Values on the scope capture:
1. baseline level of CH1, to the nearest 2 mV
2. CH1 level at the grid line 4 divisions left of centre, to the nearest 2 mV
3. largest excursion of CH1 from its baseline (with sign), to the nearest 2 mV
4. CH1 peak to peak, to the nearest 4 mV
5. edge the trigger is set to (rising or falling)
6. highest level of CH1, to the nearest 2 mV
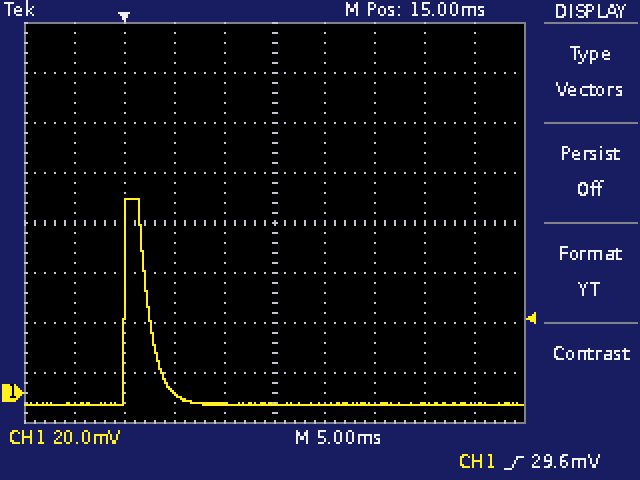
-4 mV
-4 mV
+82 mV
84 mV
rising
78 mV
